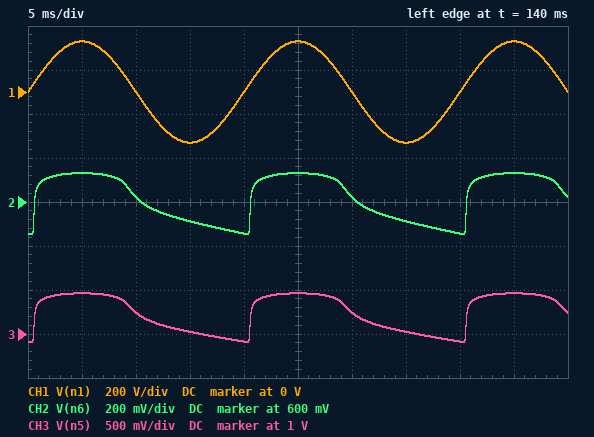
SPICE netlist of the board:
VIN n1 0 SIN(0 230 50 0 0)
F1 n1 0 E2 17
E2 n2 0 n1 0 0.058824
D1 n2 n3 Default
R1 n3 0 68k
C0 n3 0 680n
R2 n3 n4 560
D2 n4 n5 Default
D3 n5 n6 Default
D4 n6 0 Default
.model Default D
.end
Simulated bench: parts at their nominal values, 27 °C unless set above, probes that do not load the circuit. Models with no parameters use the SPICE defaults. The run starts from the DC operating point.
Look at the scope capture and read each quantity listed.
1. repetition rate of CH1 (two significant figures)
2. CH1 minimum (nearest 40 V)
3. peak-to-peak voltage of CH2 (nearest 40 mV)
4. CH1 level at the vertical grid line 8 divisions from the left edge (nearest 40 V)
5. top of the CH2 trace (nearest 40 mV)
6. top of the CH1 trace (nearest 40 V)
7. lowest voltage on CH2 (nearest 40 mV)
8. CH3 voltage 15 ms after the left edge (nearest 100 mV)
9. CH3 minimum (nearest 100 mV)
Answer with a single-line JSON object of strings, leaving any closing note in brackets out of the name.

{"repetition rate of CH1": "50 Hz", "CH1 minimum": "-240 V", "peak-to-peak voltage of CH2": "280 mV", "CH1 level at the vertical grid line 8 divisions from the left edge": "0 V", "top of the CH2 trace": "720 mV", "top of the CH1 trace": "240 V", "lowest voltage on CH2": "440 mV", "CH3 voltage 15 ms after the left edge": "1.0 V", "CH3 minimum": "900 mV"}
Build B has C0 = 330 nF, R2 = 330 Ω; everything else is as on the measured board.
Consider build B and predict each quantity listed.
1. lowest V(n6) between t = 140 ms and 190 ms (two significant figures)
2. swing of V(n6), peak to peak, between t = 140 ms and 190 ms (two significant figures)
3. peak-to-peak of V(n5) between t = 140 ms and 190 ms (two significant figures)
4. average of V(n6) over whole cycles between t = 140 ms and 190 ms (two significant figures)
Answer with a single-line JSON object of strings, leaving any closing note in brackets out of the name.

{"lowest V(n6) between t = 140 ms and 190 ms": "350 mV", "swing of V(n6), peak to peak, between t = 140 ms and 190 ms": "400 mV", "peak-to-peak of V(n5) between t = 140 ms and 190 ms": "800 mV", "average of V(n6) over whole cycles between t = 140 ms and 190 ms": "570 mV"}
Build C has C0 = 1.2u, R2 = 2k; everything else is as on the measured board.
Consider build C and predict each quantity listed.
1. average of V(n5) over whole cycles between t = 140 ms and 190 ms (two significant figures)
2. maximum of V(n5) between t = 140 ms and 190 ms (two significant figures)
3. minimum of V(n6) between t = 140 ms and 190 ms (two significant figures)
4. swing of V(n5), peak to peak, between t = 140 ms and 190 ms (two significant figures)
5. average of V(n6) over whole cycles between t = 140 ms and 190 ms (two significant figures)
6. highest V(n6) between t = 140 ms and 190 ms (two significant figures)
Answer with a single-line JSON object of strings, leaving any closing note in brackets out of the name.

{"average of V(n5) over whole cycles between t = 140 ms and 190 ms": "1.3 V", "maximum of V(n5) between t = 140 ms and 190 ms": "1.4 V", "minimum of V(n6) between t = 140 ms and 190 ms": "550 mV", "swing of V(n5), peak to peak, between t = 140 ms and 190 ms": "290 mV", "average of V(n6) over whole cycles between t = 140 ms and 190 ms": "640 mV", "highest V(n6) between t = 140 ms and 190 ms": "700 mV"}
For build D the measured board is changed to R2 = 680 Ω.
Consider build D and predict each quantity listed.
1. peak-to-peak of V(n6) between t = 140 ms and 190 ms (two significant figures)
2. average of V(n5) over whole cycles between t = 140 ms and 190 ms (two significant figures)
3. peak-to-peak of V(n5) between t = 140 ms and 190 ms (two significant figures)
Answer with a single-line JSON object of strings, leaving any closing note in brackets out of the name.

{"peak-to-peak of V(n6) between t = 140 ms and 190 ms": "270 mV", "average of V(n5) over whole cycles between t = 140 ms and 190 ms": "1.2 V", "peak-to-peak of V(n5) between t = 140 ms and 190 ms": "540 mV"}
